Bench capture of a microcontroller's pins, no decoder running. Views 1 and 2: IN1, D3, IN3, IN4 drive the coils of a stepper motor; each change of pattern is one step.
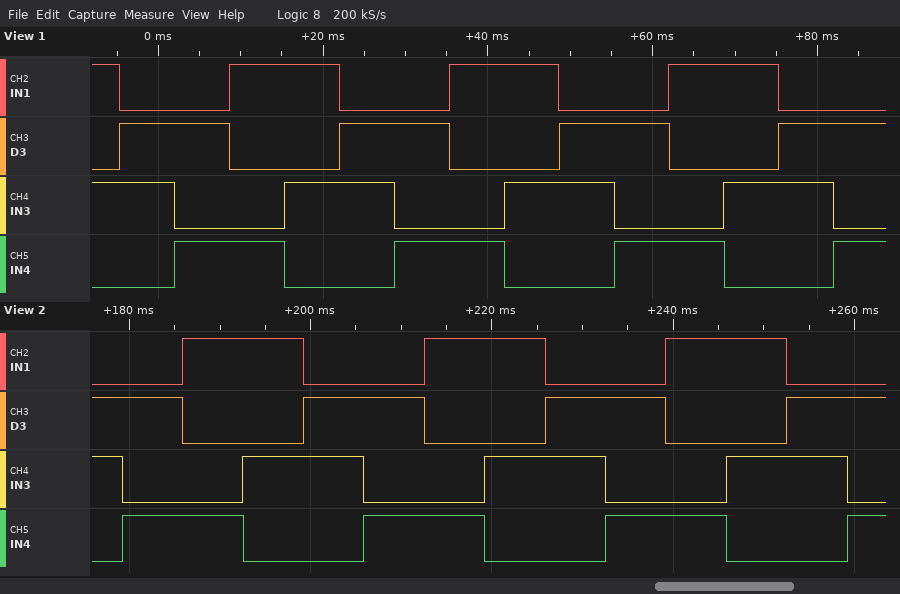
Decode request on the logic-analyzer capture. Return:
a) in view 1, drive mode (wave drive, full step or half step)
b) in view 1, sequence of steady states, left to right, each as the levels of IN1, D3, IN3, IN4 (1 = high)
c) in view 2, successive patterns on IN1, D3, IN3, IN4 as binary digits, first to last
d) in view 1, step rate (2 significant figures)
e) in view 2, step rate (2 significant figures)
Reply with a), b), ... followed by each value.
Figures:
a) full step
b) 1010 0110 0101 1001 1010 0110 0101 1001 1010 0110 0101 1001 1010 0110 0101
c) 0110 0101 1001 1010 0110 0101 1001 1010 0110 0101 1001 1010 0110 0101
d) 150 steps/s
e) 150 steps/s
